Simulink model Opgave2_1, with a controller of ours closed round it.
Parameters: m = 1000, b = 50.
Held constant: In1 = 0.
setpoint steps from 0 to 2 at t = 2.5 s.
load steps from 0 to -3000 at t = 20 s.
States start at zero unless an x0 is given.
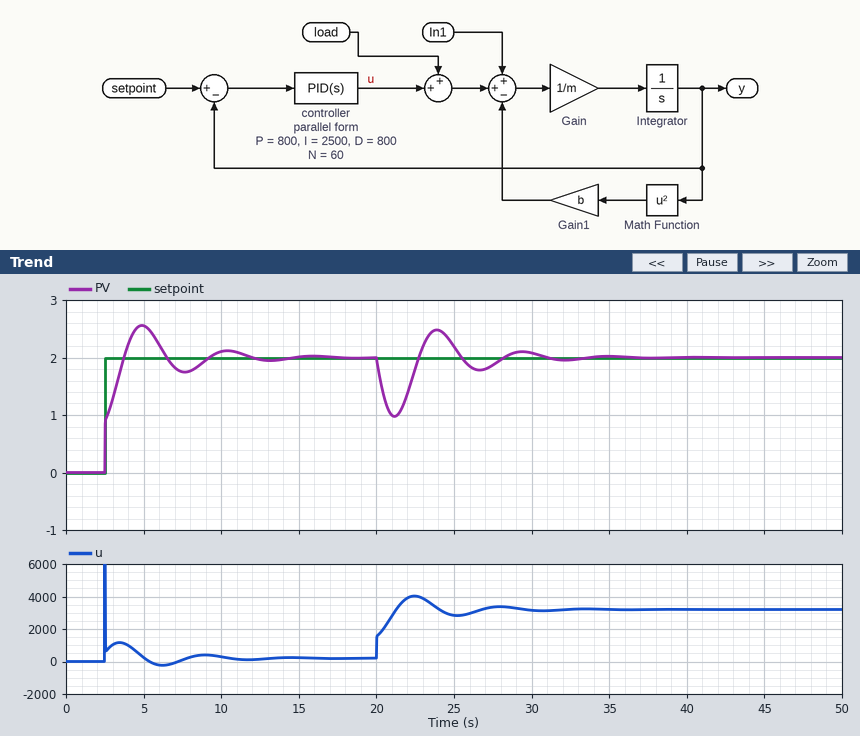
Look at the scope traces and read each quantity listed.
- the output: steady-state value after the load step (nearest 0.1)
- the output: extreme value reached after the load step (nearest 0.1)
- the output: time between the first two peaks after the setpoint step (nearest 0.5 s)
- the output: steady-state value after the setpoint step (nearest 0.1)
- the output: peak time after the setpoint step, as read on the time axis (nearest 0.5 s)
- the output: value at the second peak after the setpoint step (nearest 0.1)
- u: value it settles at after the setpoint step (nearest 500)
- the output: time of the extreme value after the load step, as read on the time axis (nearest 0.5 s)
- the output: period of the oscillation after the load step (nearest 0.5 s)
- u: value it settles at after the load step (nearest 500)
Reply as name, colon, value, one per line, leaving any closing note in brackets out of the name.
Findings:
the output: steady-state value after the load step: 2.0
the output: extreme value reached after the load step: 1.0
the output: time between the first two peaks after the setpoint step: 5.5 s
the output: steady-state value after the setpoint step: 2.0
the output: peak time after the setpoint step, as read on the time axis: 5.0 s
the output: value at the second peak after the setpoint step: 2.1
u: value it settles at after the setpoint step: 0
the output: time of the extreme value after the load step, as read on the time axis: 21.0 s
the output: period of the oscillation after the load step: 5.5 s
u: value it settles at after the load step: 3000
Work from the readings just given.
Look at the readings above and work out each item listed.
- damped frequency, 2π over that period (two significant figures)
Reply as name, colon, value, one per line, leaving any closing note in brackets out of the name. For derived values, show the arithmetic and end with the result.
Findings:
damped frequency, 2π over that period: 2π / 5.5 = 1.1 rad/s
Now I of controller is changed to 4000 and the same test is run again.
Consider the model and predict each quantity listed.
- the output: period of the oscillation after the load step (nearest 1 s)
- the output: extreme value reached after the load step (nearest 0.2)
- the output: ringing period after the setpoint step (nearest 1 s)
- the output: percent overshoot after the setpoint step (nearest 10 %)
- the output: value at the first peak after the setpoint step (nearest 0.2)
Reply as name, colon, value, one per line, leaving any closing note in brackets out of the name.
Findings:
the output: period of the oscillation after the load step: 4 s
the output: extreme value reached after the load step: 1.2
the output: ringing period after the setpoint step: 4 s
the output: percent overshoot after the setpoint step: 30 %
the output: value at the first peak after the setpoint step: 2.6
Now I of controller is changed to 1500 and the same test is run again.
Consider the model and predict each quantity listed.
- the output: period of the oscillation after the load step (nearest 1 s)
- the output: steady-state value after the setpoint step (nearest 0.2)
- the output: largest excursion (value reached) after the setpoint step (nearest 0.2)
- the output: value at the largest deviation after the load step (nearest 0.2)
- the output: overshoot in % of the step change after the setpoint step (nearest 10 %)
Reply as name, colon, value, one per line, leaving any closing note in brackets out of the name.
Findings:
the output: period of the oscillation after the load step: 7 s
the output: steady-state value after the setpoint step: 2.0
the output: largest excursion (value reached) after the setpoint step: 2.4
the output: value at the largest deviation after the load step: 0.8
the output: overshoot in % of the step change after the setpoint step: 20 %
